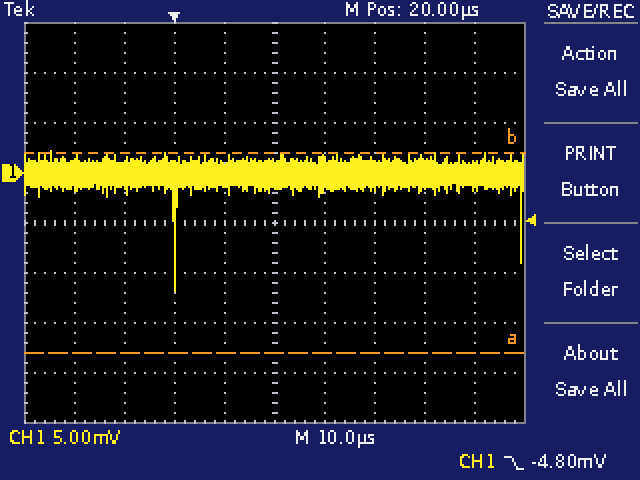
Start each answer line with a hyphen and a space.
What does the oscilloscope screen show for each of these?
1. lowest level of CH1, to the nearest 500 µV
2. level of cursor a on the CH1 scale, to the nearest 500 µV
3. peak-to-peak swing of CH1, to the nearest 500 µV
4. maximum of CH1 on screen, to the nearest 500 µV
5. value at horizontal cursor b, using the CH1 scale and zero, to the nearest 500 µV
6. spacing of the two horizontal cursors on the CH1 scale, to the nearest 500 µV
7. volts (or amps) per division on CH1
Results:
- -12.0 mV
- -18.0 mV
- 14.0 mV
- 2.0 mV
- 2.0 mV
- 20.0 mV
- 5 mV
